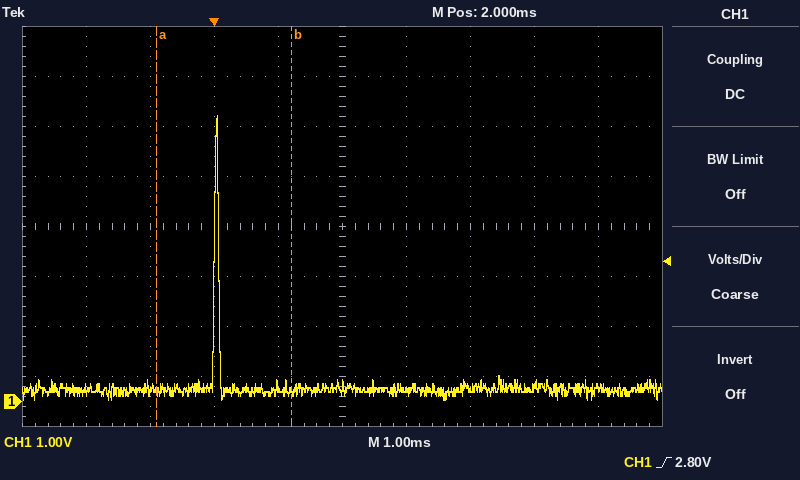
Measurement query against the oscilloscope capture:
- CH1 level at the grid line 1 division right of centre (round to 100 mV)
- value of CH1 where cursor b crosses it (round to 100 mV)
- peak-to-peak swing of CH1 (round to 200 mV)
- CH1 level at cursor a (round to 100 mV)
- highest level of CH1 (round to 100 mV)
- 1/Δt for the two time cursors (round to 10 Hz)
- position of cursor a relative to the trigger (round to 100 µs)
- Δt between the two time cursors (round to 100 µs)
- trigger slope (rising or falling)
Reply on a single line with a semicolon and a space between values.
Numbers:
200 mV; 200 mV; 5.6 V; 200 mV; 5.7 V; 480 Hz; -900 µs; 2.1 ms; rising
